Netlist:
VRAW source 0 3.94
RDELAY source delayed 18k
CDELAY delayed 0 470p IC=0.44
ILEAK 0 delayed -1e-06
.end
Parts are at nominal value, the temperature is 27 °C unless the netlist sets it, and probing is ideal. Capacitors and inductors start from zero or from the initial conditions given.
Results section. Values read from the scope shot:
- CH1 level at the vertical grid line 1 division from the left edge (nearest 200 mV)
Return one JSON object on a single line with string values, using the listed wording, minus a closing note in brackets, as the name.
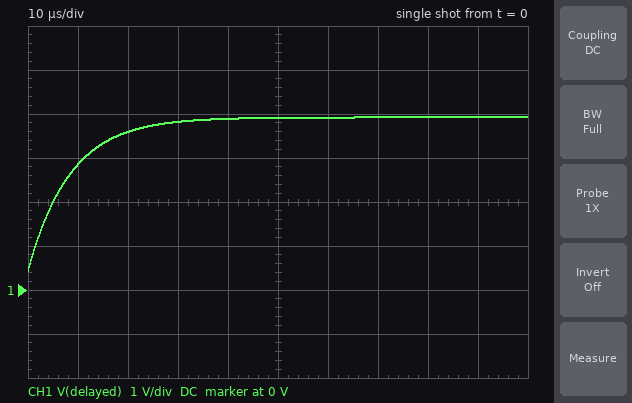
{"CH1 level at the vertical grid line 1 division from the left edge": "2.8 V"}
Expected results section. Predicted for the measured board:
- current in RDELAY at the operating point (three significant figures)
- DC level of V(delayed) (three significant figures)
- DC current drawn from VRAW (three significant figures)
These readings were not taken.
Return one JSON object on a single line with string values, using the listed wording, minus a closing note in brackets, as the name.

{"current in RDELAY at the operating point": "1.00 µA", "DC level of V(delayed)": "3.92 V", "DC current drawn from VRAW": "1.00 µA"}
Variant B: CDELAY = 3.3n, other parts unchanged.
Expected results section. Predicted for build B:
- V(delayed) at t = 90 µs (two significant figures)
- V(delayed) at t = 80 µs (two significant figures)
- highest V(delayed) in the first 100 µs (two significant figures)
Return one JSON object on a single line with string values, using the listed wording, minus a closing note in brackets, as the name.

{"V(delayed) at t = 90 µs": "3.2 V", "V(delayed) at t = 80 µs": "3.0 V", "highest V(delayed) in the first 100 µs": "3.3 V"}
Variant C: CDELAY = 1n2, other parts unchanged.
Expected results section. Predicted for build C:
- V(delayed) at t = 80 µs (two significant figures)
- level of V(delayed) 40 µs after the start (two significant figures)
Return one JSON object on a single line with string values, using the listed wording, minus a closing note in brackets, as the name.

{"V(delayed) at t = 80 µs": "3.8 V", "level of V(delayed) 40 µs after the start": "3.4 V"}
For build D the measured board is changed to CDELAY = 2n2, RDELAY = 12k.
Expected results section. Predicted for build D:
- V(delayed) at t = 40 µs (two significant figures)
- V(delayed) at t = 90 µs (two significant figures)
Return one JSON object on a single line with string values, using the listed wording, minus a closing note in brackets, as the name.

{"V(delayed) at t = 40 µs": "3.2 V", "V(delayed) at t = 90 µs": "3.8 V"}
